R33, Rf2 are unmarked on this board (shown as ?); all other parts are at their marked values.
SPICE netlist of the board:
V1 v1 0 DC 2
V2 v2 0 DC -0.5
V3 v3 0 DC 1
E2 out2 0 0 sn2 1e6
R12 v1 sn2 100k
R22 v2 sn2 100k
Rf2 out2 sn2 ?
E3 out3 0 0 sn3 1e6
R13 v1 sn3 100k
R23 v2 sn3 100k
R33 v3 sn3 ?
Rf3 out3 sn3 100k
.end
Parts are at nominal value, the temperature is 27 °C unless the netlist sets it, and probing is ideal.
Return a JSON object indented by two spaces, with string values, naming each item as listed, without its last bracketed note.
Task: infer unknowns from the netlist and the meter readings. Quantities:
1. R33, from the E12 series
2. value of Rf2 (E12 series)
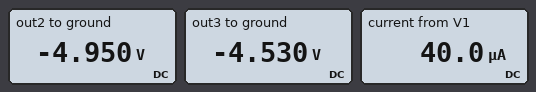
{
  "R33, from the E12 series": "33 kΩ",
  "value of Rf2": "330 kΩ"
}
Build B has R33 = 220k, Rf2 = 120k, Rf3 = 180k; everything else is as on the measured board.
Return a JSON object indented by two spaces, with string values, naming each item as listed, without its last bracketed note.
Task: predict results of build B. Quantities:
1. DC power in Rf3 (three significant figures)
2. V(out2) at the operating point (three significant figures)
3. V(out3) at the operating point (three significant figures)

{
  "DC power in Rf3": "68.8 µW",
  "V(out2) at the operating point": "-1.80 V",
  "V(out3) at the operating point": "-3.52 V"
}
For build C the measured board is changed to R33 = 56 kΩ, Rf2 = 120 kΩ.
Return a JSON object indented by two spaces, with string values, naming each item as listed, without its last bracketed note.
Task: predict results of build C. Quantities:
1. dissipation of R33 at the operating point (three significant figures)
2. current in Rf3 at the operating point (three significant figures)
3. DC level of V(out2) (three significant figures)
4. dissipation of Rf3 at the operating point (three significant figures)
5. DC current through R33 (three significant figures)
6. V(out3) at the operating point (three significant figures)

{
  "dissipation of R33 at the operating point": "17.9 µW",
  "current in Rf3 at the operating point": "32.9 µA",
  "DC level of V(out2)": "-1.80 V",
  "dissipation of Rf3 at the operating point": "108 µW",
  "DC current through R33": "17.9 µA",
  "V(out3) at the operating point": "-3.29 V"
}
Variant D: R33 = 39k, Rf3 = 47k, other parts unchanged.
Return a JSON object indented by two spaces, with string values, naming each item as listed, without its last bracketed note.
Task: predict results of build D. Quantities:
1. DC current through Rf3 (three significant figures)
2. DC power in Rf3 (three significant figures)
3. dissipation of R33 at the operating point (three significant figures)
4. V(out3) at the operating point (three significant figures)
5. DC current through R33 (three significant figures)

{
  "DC current through Rf3": "40.6 µA",
  "DC power in Rf3": "77.6 µW",
  "dissipation of R33 at the operating point": "25.6 µW",
  "V(out3) at the operating point": "-1.91 V",
  "DC current through R33": "25.6 µA"
}
